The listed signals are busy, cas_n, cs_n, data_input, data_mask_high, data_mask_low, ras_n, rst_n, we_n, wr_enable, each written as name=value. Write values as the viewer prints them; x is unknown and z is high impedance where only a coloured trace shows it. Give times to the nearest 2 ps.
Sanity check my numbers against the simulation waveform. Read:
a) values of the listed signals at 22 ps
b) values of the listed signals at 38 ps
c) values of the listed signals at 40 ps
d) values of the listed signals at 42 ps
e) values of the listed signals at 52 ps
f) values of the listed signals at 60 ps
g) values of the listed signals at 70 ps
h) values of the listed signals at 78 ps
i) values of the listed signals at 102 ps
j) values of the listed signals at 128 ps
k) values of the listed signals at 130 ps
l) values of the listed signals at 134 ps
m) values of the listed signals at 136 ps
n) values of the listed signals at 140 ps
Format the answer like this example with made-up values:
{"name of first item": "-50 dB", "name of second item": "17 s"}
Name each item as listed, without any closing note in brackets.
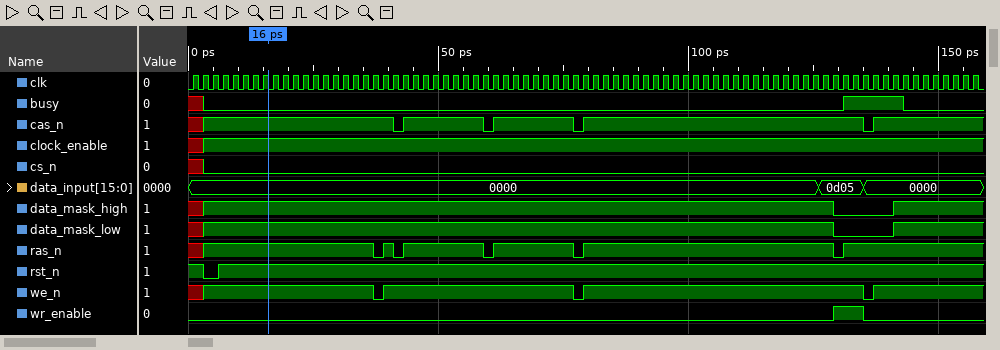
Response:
{"values of the listed signals at 22 ps": "busy=0, cas_n=1, cs_n=0, data_input=0000, data_mask_high=1, data_mask_low=1, ras_n=1, rst_n=1, we_n=1, wr_enable=0", "values of the listed signals at 38 ps": "busy=0, cas_n=1, cs_n=0, data_input=0000, data_mask_high=1, data_mask_low=1, ras_n=0, rst_n=1, we_n=0, wr_enable=0", "values of the listed signals at 40 ps": "busy=0, cas_n=1, cs_n=0, data_input=0000, data_mask_high=1, data_mask_low=1, ras_n=1, rst_n=1, we_n=1, wr_enable=0", "values of the listed signals at 42 ps": "busy=0, cas_n=0, cs_n=0, data_input=0000, data_mask_high=1, data_mask_low=1, ras_n=0, rst_n=1, we_n=1, wr_enable=0", "values of the listed signals at 52 ps": "busy=0, cas_n=1, cs_n=0, data_input=0000, data_mask_high=1, data_mask_low=1, ras_n=1, rst_n=1, we_n=1, wr_enable=0", "values of the listed signals at 60 ps": "busy=0, cas_n=0, cs_n=0, data_input=0000, data_mask_high=1, data_mask_low=1, ras_n=0, rst_n=1, we_n=1, wr_enable=0", "values of the listed signals at 70 ps": "busy=0, cas_n=1, cs_n=0, data_input=0000, data_mask_high=1, data_mask_low=1, ras_n=1, rst_n=1, we_n=1, wr_enable=0", "values of the listed signals at 78 ps": "busy=0, cas_n=0, cs_n=0, data_input=0000, data_mask_high=1, data_mask_low=1, ras_n=0, rst_n=1, we_n=0, wr_enable=0", "values of the listed signals at 102 ps": "busy=0, cas_n=1, cs_n=0, data_input=0000, data_mask_high=1, data_mask_low=1, ras_n=1, rst_n=1, we_n=1, wr_enable=0", "values of the listed signals at 128 ps": "busy=0, cas_n=1, cs_n=0, data_input=0d05, data_mask_high=1, data_mask_low=1, ras_n=1, rst_n=1, we_n=1, wr_enable=0", "values of the listed signals at 130 ps": "busy=0, cas_n=1, cs_n=0, data_input=0d05, data_mask_high=0, data_mask_low=0, ras_n=0, rst_n=1, we_n=1, wr_enable=1", "values of the listed signals at 134 ps": "busy=1, cas_n=1, cs_n=0, data_input=0d05, data_mask_high=0, data_mask_low=0, ras_n=1, rst_n=1, we_n=1, wr_enable=1", "values of the listed signals at 136 ps": "busy=1, cas_n=0, cs_n=0, data_input=0000, data_mask_high=0, data_mask_low=0, ras_n=1, rst_n=1, we_n=0, wr_enable=0", "values of the listed signals at 140 ps": "busy=1, cas_n=1, cs_n=0, data_input=0000, data_mask_high=0, data_mask_low=0, ras_n=1, rst_n=1, we_n=1, wr_enable=0"}
